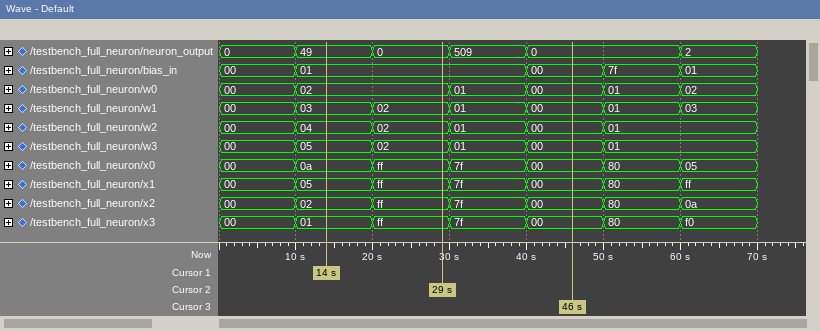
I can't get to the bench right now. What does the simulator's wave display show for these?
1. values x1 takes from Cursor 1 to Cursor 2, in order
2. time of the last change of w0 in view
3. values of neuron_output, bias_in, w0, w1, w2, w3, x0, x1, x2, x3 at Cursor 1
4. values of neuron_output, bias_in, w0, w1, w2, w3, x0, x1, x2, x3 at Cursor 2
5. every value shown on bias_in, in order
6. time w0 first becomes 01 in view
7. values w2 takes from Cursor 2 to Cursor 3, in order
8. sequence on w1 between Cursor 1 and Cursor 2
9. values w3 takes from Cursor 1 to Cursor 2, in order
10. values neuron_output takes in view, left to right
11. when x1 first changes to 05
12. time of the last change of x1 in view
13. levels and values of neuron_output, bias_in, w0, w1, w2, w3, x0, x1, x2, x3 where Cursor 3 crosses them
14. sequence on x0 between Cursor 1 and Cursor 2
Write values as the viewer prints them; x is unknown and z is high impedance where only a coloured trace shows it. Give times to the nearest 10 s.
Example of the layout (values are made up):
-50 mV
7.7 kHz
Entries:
05, ff
60 s
neuron_output=49, bias_in=01, w0=02, w1=03, w2=04, w3=05, x0=0a, x1=05, x2=02, x3=01
neuron_output=0, bias_in=01, w0=02, w1=02, w2=02, w3=02, x0=ff, x1=ff, x2=ff, x3=ff
00, 01, 00, 7f, 01
30 s
02, 01, 00
03, 02
05, 02
0, 49, 0, 509, 0, 2
10 s
60 s
neuron_output=0, bias_in=00, w0=00, w1=00, w2=00, w3=00, x0=00, x1=00, x2=00, x3=00
0a, ff
